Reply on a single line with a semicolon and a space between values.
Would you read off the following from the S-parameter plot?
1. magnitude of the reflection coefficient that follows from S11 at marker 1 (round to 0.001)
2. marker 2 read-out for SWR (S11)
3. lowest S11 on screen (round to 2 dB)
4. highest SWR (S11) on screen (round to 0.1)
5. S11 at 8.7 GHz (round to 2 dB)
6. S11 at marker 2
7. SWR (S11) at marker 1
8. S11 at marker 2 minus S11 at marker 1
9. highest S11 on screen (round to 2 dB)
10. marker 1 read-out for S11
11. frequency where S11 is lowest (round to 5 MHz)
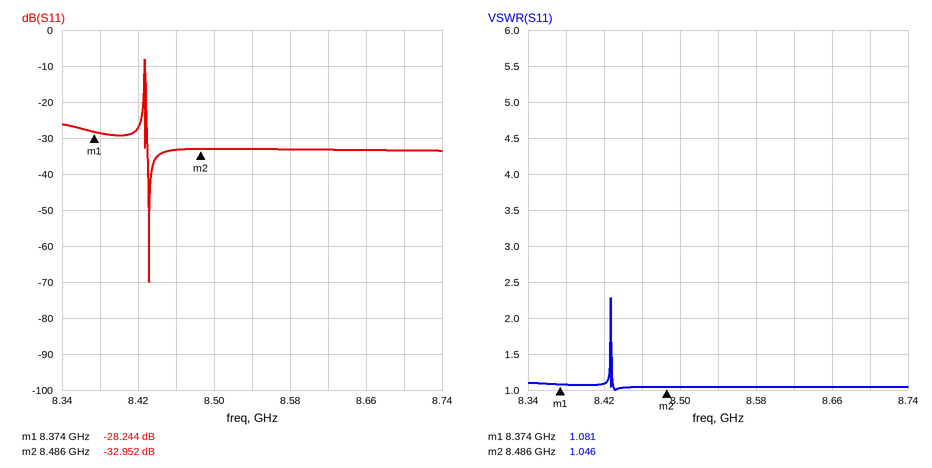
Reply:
0.039; 1.046; -70 dB; 2.3; -34 dB; -32.952 dB; 1.081; -4.708 dB; -8 dB; -28.244 dB; 8.430 GHz
